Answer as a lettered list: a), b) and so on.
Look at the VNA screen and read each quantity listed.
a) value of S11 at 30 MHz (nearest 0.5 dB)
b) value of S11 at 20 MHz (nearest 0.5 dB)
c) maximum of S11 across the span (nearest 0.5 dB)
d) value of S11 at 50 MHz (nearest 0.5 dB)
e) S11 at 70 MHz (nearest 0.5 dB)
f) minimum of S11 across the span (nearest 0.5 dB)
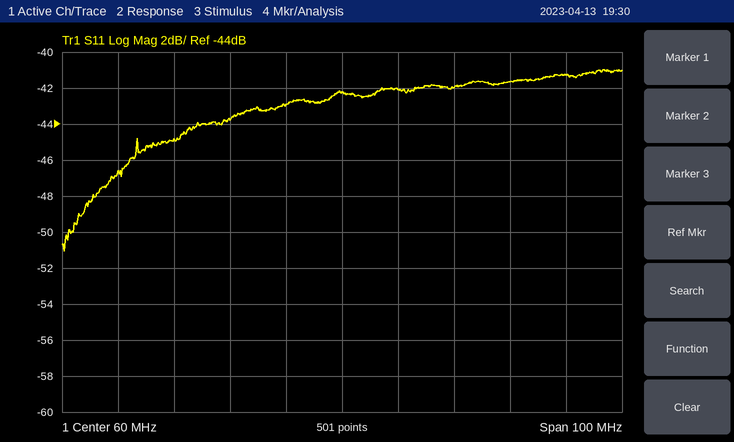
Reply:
a) -45.0 dB
b) -46.5 dB
c) -41.0 dB
d) -43.0 dB
e) -42.0 dB
f) -51.0 dB
